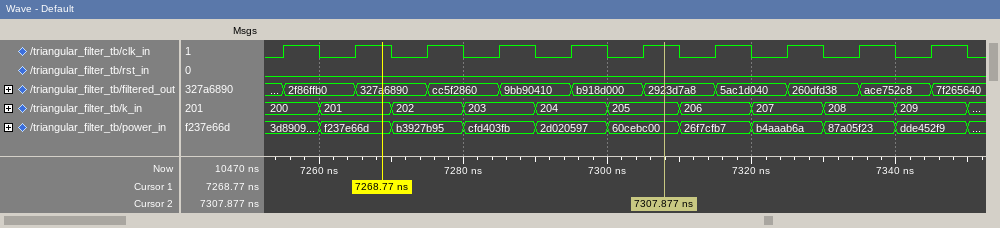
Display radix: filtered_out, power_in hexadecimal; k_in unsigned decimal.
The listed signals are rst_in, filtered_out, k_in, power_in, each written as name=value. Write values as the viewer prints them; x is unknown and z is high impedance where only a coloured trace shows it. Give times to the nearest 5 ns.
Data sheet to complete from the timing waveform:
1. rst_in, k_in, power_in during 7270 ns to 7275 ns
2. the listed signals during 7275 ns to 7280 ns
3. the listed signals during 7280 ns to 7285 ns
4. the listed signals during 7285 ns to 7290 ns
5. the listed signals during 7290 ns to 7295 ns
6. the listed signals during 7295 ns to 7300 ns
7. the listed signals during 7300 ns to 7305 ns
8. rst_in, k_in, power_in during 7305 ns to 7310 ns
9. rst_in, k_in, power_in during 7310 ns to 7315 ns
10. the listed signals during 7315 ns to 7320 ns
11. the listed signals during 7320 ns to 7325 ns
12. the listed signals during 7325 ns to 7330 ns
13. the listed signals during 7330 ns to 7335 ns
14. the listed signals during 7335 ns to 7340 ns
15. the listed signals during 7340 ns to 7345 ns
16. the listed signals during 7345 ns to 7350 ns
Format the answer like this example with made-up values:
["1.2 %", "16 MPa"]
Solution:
["rst_in=0, k_in=202, power_in=b3927b95", "rst_in=0, filtered_out=cc5f2860, k_in=202, power_in=b3927b95", "rst_in=0, filtered_out=cc5f2860, k_in=203, power_in=cfd403fb", "rst_in=0, filtered_out=9bb90410, k_in=203, power_in=cfd403fb", "rst_in=0, filtered_out=9bb90410, k_in=204, power_in=2d020597", "rst_in=0, filtered_out=b918d000, k_in=204, power_in=2d020597", "rst_in=0, filtered_out=b918d000, k_in=205, power_in=60cebc00", "rst_in=0, k_in=205, power_in=60cebc00", "rst_in=0, k_in=206, power_in=26f7cfb7", "rst_in=0, filtered_out=5ac1d040, k_in=206, power_in=26f7cfb7", "rst_in=0, filtered_out=5ac1d040, k_in=207, power_in=b4aaab6a", "rst_in=0, filtered_out=260dfd38, k_in=207, power_in=b4aaab6a", "rst_in=0, filtered_out=260dfd38, k_in=208, power_in=87a05f23", "rst_in=0, filtered_out=ace752c8, k_in=208, power_in=87a05f23", "rst_in=0, filtered_out=ace752c8, k_in=209, power_in=dde452f9", "rst_in=0, filtered_out=7f265640, k_in=209, power_in=dde452f9"]
